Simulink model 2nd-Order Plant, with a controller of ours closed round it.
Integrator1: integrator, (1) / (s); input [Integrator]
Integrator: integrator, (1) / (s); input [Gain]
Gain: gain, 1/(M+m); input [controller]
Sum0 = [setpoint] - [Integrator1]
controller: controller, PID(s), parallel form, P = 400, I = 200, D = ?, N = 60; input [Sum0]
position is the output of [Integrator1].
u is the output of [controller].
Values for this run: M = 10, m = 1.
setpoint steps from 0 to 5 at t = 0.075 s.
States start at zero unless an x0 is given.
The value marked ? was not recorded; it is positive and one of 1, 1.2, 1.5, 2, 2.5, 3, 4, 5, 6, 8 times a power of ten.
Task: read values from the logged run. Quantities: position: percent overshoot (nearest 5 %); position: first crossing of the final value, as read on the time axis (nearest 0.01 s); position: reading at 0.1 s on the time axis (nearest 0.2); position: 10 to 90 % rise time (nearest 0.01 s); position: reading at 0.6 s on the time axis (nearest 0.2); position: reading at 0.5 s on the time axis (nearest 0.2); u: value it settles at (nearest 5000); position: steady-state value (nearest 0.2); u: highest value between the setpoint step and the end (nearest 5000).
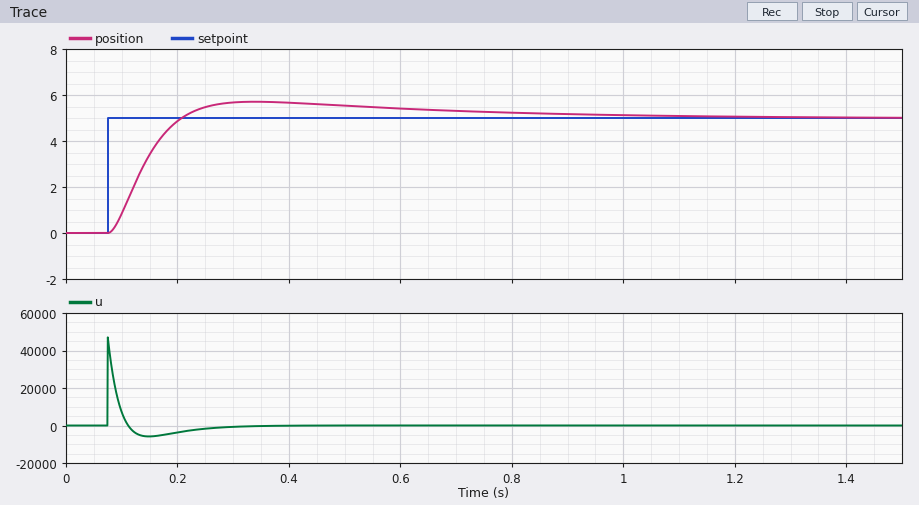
15 %
0.21 s
0.8
0.09 s
5.4
5.6
0
5.0
45000
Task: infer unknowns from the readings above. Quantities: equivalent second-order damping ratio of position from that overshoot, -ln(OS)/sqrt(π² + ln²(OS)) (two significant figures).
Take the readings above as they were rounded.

0.52
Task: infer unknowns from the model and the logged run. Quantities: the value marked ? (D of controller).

150
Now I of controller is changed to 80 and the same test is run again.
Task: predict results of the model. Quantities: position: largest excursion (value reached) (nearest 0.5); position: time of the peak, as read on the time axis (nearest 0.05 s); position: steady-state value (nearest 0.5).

5.5
0.35 s
5.0
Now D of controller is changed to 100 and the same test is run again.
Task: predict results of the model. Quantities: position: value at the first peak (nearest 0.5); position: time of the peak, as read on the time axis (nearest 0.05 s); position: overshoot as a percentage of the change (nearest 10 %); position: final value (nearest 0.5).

6.0
0.40 s
20 %
5.0
